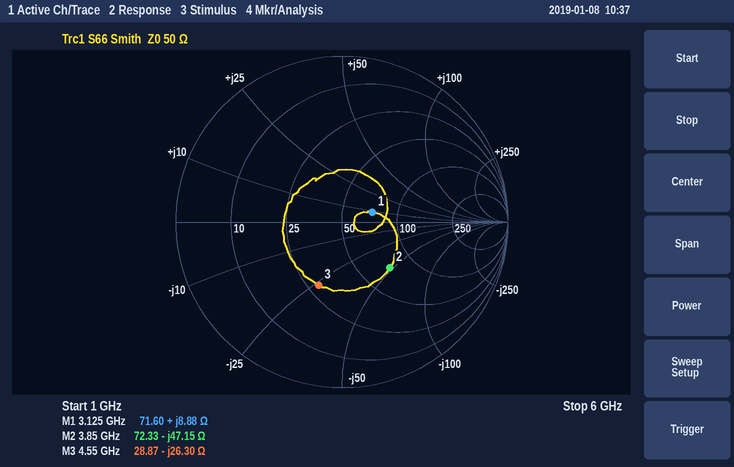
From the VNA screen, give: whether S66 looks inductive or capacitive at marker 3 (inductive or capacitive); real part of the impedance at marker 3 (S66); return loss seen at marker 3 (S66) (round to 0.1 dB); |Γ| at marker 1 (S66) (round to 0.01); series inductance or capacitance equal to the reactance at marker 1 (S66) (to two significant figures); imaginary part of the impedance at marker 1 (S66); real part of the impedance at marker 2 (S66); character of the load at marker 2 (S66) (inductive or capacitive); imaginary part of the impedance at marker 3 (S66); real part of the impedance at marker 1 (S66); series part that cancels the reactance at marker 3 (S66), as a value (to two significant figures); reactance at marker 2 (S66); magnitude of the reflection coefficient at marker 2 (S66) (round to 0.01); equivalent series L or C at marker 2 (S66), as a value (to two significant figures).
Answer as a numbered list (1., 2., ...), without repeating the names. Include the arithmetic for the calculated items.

1. capacitive
2. 28.87 Ω
3. 7.8 dB
4. 0.19
5. L = 8.88 Ω/(2π × 3.125 GHz) ≈ 452 pH, so 450 pH to two significant figures
6. +8.88 Ω
7. 72.33 Ω
8. capacitive
9. -26.30 Ω
10. 71.60 Ω
11. L = 26.3 Ω/(2π × 4.55 GHz) ≈ 920 pH
12. -47.15 Ω
13. 0.40
14. C = 1/(2π × 3.85 GHz × 47.15 Ω) ≈ 877 fF, so 880 fF to two significant figures
